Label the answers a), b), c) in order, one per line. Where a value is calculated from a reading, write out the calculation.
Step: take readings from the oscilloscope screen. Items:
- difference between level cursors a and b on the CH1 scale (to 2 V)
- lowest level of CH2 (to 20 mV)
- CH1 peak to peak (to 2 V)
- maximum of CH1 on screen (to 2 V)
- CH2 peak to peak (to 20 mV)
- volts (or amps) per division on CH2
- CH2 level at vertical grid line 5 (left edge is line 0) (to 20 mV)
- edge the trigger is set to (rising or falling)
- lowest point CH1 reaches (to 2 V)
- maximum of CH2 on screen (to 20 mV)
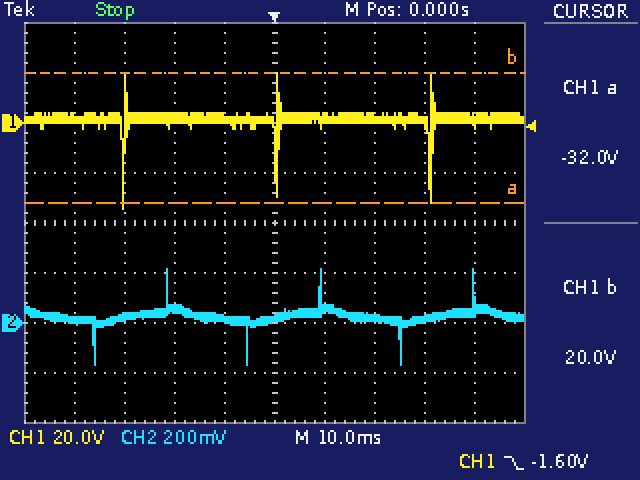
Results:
a) 52 V
b) -160 mV
c) 20 V − (-34 V) = 54 V
d) 20 V
e) 220 mV − (-160 mV) = 380 mV
f) 200 mV
g) 20 mV
h) falling
i) -34 V
j) 220 mV
